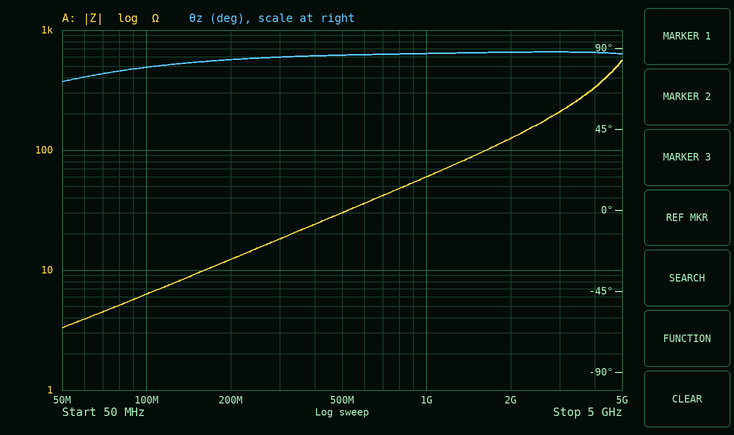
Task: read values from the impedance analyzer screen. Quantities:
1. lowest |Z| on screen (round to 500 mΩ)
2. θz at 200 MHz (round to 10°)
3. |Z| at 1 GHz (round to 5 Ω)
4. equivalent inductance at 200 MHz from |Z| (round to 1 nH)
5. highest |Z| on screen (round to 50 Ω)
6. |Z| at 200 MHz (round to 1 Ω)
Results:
3.5 Ω
80°
60 Ω
10 nH
550 Ω
12 Ω
